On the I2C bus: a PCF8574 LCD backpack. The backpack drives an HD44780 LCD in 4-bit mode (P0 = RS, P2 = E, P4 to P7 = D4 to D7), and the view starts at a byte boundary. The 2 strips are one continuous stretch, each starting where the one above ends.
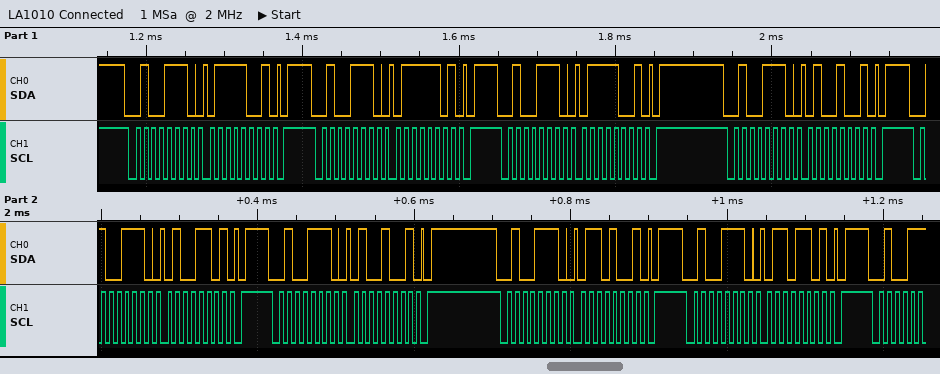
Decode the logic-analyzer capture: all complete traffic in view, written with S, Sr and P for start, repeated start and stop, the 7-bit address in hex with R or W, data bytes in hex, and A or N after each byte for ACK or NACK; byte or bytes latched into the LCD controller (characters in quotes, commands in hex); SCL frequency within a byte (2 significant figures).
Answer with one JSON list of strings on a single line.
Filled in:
["S 27W A 79 A P S 27W A 7D A P S 27W A 79 A P S 27W A 49 A P S 27W A 4D A P S 27W A 49 A P S 27W A 69 A P S 27W A 6D A P", "'t'", "100 kHz"]
